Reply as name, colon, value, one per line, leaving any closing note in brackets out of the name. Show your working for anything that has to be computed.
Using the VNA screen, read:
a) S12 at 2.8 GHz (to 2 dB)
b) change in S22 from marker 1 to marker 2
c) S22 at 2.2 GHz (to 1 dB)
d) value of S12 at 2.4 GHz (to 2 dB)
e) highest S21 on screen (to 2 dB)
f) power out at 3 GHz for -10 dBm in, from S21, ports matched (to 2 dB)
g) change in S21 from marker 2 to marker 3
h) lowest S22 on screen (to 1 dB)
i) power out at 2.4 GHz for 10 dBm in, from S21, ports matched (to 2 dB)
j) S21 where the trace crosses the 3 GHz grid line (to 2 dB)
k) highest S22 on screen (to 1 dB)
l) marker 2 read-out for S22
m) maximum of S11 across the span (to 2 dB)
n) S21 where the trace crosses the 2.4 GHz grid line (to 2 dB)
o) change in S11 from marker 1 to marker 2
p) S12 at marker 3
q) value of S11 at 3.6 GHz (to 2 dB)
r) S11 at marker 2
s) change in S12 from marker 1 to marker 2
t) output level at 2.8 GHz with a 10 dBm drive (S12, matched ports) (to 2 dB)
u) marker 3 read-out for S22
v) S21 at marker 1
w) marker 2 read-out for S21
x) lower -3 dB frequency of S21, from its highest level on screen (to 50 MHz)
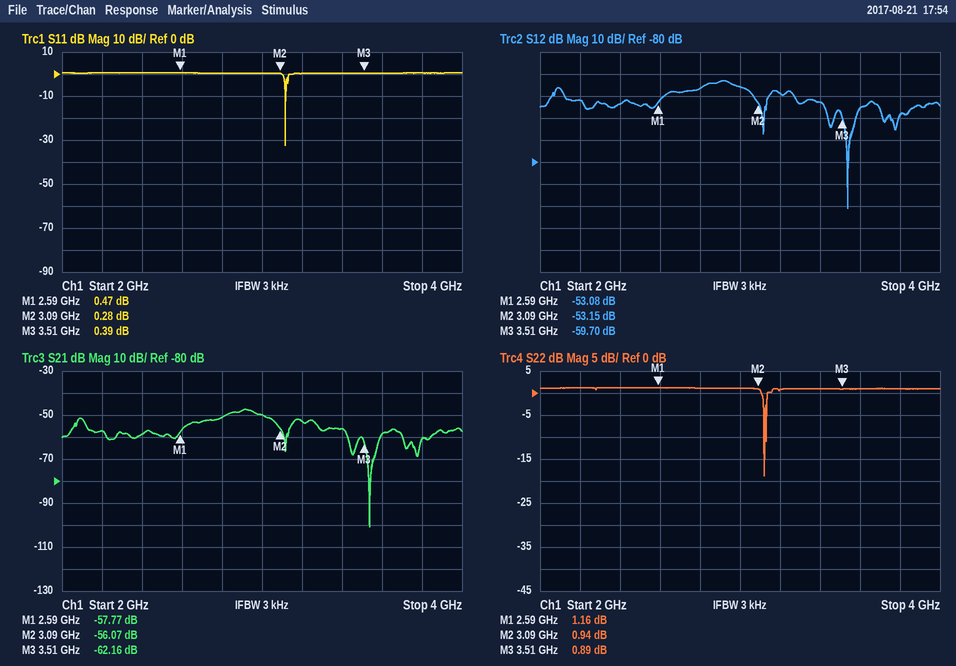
S12 at 2.8 GHz: -46 dB
change in S22 from marker 1 to marker 2: 0.94 − (1.16) = -0.22 dB
S22 at 2.2 GHz: 1 dB
value of S12 at 2.4 GHz: -54 dB
highest S21 on screen: -48 dB
power out at 3 GHz for -10 dBm in, from S21, ports matched: -10 dBm + (-50 dB) = -60 dBm
change in S21 from marker 2 to marker 3: -62.16 − (-56.07) = -6.09 dB
lowest S22 on screen: -19 dB
power out at 2.4 GHz for 10 dBm in, from S21, ports matched: 10 dBm + (-58 dB) = -48 dBm
S21 where the trace crosses the 3 GHz grid line: -50 dB
highest S22 on screen: 1 dB
marker 2 read-out for S22: 0.94 dB
maximum of S11 across the span: 0 dB
S21 where the trace crosses the 2.4 GHz grid line: -58 dB
change in S11 from marker 1 to marker 2: 0.28 − (0.47) = -0.19 dB
S12 at marker 3: -59.70 dB
value of S11 at 3.6 GHz: 0 dB
S11 at marker 2: 0.28 dB
change in S12 from marker 1 to marker 2: -53.15 − (-53.08) = -0.07 dB
output level at 2.8 GHz with a 10 dBm drive (S12, matched ports): 10 dBm + (-46 dB) = -36 dBm
marker 3 read-out for S22: 0.89 dB
S21 at marker 1: -57.77 dB
marker 2 read-out for S21: -56.07 dB
lower -3 dB frequency of S21, from its highest level on screen: 2.80 GHz
